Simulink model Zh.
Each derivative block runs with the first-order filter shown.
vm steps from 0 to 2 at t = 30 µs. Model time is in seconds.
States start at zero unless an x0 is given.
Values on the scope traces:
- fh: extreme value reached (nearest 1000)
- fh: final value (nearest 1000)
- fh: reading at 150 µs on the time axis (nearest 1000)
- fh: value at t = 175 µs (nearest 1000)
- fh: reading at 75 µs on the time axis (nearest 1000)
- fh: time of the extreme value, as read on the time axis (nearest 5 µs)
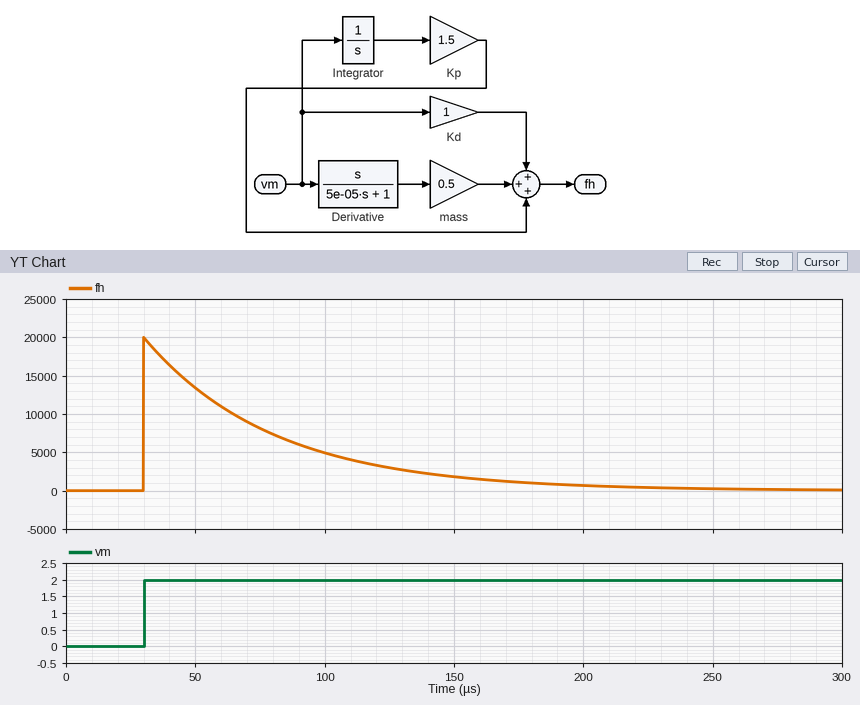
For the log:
20000
0
2000
1000
8000
30 µs
